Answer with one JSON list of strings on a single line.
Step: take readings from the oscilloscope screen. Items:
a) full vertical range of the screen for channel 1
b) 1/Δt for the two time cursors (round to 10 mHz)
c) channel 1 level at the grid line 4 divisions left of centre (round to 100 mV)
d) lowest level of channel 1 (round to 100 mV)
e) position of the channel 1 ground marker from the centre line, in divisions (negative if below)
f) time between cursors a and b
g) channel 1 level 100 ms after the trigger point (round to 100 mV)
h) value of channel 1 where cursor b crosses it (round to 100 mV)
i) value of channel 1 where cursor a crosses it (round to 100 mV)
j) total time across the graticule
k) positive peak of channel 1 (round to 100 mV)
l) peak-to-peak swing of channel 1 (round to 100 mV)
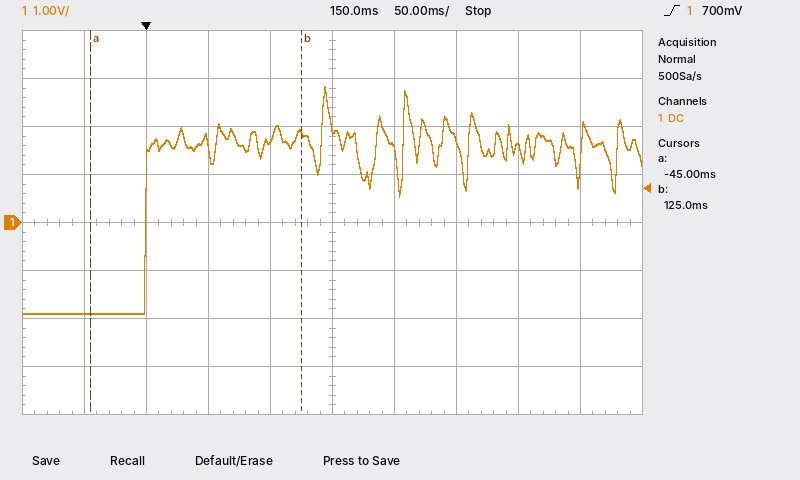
["8 V", "5.88 Hz", "-1.9 V", "-1.9 V", "0.0 div", "170 ms", "1.7 V", "1.9 V", "-1.9 V", "500 ms", "2.8 V", "4.7 V"]
